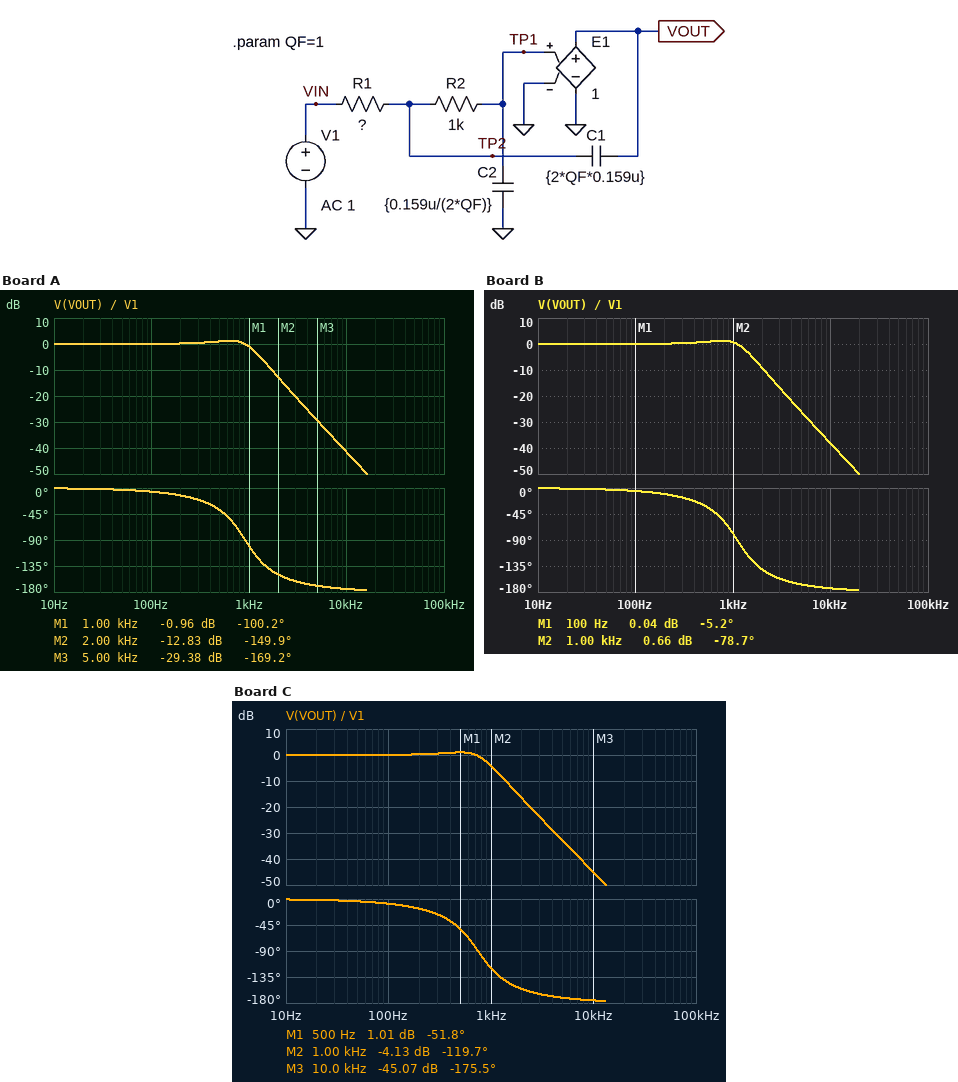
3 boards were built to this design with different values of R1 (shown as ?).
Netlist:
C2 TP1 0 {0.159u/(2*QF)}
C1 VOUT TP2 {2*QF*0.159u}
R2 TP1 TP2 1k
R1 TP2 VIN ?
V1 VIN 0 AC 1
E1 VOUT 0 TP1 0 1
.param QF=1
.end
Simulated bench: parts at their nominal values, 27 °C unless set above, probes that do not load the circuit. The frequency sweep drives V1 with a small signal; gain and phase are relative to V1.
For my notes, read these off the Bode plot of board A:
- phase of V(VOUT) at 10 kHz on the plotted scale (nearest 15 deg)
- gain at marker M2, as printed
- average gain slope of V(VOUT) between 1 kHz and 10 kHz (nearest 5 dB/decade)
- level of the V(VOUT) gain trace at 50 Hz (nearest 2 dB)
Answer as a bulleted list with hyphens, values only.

- -180 deg
- -12.83 dB
- -40 dB/decade
- 0 dB
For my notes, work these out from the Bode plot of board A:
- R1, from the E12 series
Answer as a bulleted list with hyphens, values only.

- 1.2 kΩ
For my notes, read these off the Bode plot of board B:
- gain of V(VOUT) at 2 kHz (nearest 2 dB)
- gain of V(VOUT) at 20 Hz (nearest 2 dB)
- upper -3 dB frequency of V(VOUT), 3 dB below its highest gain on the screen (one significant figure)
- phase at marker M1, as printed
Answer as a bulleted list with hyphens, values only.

- -10 dB
- 0 dB
- 1 kHz
- -5.2 deg
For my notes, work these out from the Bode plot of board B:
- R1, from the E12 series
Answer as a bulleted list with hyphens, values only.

- 820 Ω
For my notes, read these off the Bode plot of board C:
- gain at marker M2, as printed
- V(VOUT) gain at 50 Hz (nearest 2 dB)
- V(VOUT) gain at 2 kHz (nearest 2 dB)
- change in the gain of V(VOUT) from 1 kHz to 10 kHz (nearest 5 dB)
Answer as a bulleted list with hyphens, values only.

- -4.13 dB
- 0 dB
- -16 dB
- -40 dB
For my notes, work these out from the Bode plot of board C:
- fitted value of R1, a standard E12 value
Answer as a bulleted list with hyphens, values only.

- 1.8 kΩ
